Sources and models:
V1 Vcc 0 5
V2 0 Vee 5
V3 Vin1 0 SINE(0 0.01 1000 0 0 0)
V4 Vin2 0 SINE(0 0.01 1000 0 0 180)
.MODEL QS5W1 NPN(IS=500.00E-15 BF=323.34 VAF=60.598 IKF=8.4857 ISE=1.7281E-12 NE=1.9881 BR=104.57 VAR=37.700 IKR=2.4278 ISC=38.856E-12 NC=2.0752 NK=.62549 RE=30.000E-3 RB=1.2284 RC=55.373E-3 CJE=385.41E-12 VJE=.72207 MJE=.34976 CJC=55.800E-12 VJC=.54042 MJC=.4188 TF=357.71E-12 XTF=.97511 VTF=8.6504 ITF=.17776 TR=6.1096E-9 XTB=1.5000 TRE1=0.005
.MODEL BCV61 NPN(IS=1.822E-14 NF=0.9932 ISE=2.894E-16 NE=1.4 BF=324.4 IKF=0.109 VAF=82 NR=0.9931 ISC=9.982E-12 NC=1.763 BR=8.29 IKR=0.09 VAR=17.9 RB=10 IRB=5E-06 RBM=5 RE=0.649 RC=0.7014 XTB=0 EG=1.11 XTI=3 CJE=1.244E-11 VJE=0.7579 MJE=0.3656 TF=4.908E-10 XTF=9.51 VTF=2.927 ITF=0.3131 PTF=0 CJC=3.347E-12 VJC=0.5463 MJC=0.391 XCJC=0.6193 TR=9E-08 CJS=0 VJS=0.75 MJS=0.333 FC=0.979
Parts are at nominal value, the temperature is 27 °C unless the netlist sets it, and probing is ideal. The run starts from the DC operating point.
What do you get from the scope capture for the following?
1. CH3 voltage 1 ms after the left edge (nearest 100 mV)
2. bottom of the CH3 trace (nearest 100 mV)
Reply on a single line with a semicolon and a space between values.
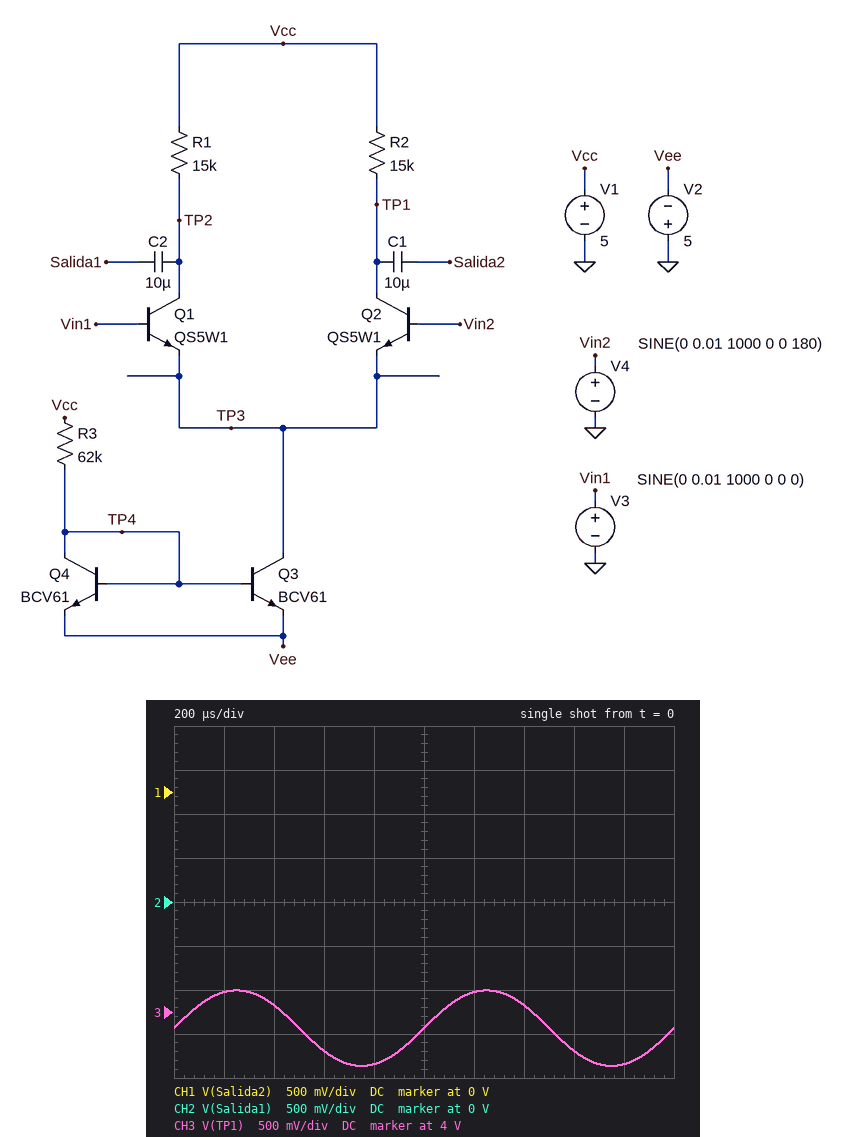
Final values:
3.8 V; 3.4 V
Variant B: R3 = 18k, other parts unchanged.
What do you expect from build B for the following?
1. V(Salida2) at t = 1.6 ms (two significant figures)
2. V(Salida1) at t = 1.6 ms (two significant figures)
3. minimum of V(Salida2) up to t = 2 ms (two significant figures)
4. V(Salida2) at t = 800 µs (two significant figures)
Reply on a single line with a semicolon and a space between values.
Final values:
97 mV; 1.8 V; -420 mV; -390 mV
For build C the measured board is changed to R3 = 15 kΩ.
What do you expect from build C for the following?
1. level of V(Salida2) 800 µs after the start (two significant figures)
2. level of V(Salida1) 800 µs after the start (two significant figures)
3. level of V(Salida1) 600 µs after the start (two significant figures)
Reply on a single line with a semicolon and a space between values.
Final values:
-500 mV; 820 mV; 770 mV
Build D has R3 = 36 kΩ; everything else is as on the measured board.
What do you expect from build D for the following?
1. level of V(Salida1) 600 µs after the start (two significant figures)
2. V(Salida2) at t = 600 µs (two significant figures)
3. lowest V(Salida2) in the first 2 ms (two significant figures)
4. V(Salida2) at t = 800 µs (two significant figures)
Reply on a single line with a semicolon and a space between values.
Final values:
3.4 V; 2.5 V; 2.2 V; 2.3 V
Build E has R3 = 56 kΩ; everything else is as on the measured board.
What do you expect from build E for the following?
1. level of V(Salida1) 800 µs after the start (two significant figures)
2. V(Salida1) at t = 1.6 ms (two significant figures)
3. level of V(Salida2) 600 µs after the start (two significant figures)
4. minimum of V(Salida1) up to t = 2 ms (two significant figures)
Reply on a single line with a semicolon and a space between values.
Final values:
4.1 V; 4.0 V; 3.4 V; 3.2 V
